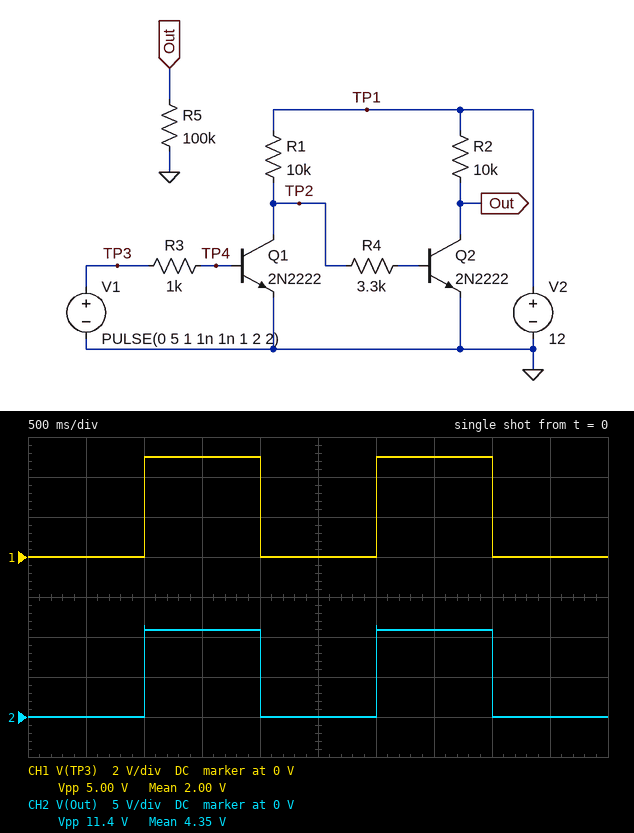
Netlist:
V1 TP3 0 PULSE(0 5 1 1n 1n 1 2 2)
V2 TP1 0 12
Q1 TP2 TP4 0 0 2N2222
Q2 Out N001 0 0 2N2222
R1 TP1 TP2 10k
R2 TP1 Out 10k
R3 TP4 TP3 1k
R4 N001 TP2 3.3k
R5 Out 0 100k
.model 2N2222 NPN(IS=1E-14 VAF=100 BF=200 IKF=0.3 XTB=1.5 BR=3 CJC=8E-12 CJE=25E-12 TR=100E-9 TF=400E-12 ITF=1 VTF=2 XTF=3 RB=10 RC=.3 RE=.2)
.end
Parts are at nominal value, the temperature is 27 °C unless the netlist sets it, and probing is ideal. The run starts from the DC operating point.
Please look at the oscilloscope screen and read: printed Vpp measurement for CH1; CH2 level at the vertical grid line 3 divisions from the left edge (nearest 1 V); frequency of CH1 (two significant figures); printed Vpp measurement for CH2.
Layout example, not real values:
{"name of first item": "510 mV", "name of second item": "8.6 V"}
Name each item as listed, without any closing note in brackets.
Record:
{"printed Vpp measurement for CH1": "5.00 V", "CH2 level at the vertical grid line 3 divisions from the left edge": "11 V", "frequency of CH1": "500 mHz", "printed Vpp measurement for CH2": "11.4 V"}
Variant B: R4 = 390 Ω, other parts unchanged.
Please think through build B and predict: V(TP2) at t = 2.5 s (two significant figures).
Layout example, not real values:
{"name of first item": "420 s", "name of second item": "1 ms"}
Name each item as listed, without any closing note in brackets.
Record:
{"V(TP2) at t = 2.5 s": "1.1 V"}
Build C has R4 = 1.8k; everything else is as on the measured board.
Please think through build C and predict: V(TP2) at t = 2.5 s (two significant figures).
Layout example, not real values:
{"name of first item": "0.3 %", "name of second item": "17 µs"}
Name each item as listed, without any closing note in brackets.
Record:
{"V(TP2) at t = 2.5 s": "2.4 V"}
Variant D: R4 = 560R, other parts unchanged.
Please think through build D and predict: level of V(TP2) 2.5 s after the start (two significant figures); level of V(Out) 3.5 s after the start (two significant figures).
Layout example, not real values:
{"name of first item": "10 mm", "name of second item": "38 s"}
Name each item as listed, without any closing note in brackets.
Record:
{"level of V(TP2) 2.5 s after the start": "1.3 V", "level of V(Out) 3.5 s after the start": "11 V"}
